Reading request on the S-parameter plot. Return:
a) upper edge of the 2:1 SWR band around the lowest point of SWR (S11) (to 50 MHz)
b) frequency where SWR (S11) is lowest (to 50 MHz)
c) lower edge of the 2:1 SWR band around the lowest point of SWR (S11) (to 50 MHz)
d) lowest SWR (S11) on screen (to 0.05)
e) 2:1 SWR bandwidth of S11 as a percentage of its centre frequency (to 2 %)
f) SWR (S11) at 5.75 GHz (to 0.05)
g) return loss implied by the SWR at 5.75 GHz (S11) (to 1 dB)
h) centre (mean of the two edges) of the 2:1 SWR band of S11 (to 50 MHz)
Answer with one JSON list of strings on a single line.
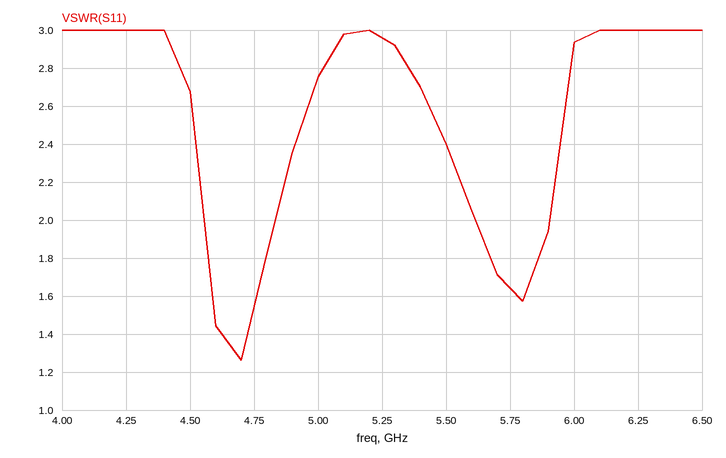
["4.85 GHz", "4.70 GHz", "4.55 GHz", "1.25", "6 %", "1.65", "12 dB", "4.70 GHz"]
